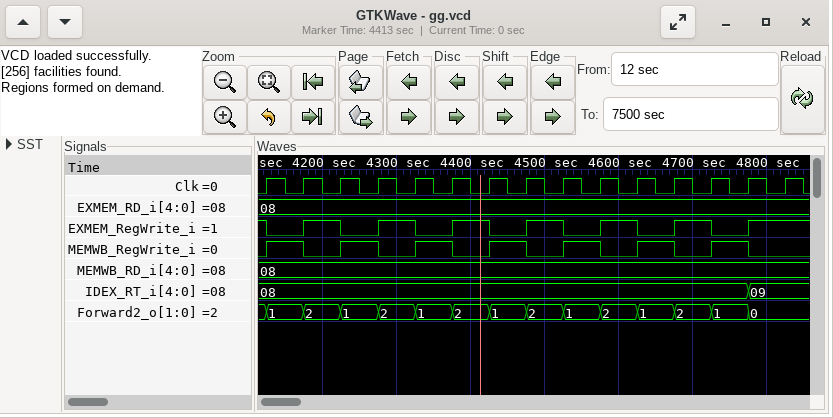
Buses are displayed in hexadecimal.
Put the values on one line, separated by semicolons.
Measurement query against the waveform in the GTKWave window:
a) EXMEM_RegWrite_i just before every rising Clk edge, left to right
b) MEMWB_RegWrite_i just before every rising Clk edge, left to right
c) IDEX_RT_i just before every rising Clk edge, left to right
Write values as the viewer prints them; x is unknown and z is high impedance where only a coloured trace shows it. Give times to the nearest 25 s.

1 0 1 0 1 0 1 0 1 0 1 0 1 0 1; 0 1 0 1 0 1 0 1 0 1 0 1 0 1 0; 08, 08, 08, 08, 08, 08, 08, 08, 08, 08, 08, 08, 08, 08, 09
